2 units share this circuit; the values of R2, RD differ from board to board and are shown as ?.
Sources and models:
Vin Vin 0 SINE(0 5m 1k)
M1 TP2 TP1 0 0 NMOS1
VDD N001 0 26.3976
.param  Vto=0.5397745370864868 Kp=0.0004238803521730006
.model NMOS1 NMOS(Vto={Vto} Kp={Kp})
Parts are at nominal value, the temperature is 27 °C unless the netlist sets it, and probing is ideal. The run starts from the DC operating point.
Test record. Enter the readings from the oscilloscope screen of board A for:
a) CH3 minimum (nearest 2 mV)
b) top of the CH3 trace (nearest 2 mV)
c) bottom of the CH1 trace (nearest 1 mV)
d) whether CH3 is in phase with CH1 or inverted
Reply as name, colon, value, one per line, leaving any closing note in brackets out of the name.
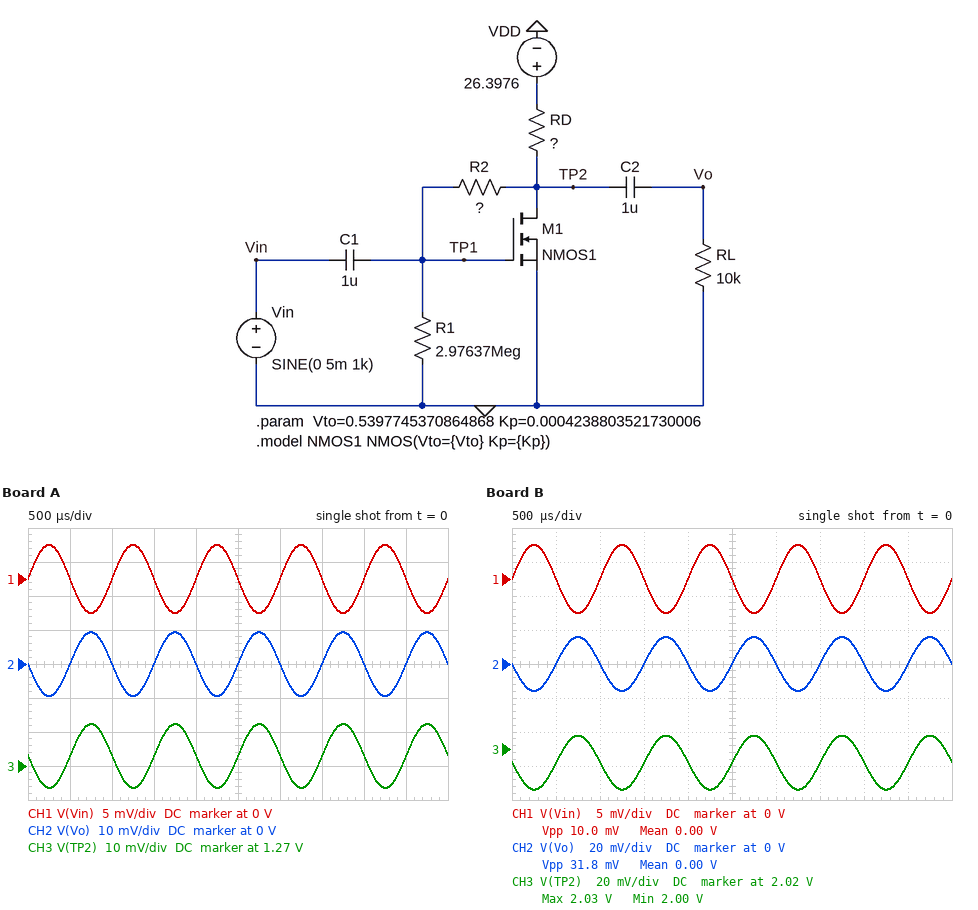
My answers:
CH3 minimum: 1.264 V
top of the CH3 trace: 1.282 V
bottom of the CH1 trace: -5 mV
whether CH3 is in phase with CH1 or inverted: inverted
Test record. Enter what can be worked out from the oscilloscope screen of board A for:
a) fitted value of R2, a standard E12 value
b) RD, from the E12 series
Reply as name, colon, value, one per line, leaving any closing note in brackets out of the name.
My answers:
fitted value of R2, a standard E12 value: 820 kΩ
RD, from the E12 series: 560 kΩ
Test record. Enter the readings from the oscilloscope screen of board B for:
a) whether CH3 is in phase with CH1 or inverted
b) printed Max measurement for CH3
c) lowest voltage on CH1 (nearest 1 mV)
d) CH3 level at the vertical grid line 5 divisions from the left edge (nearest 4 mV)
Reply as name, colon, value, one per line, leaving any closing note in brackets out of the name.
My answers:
whether CH3 is in phase with CH1 or inverted: inverted
printed Max measurement for CH3: 2.03 V
lowest voltage on CH1: -5 mV
CH3 level at the vertical grid line 5 divisions from the left edge: 2.012 V
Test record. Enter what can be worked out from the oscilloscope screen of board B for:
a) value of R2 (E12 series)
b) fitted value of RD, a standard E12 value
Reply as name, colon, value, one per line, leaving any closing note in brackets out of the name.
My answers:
value of R2: 1.5 MΩ
fitted value of RD, a standard E12 value: 180 kΩ
